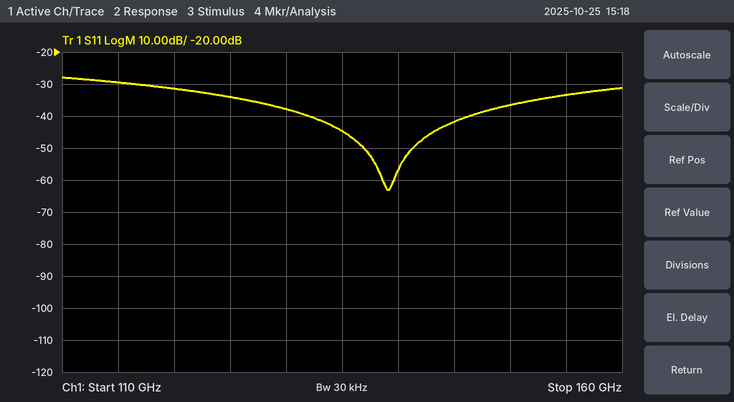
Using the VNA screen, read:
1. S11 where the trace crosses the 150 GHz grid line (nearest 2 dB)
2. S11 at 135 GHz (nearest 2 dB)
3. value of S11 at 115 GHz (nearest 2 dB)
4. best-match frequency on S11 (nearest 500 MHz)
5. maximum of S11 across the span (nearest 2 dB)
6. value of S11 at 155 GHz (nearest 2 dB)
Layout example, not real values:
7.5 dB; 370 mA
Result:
-36 dB; -44 dB; -30 dB; 139.0 GHz; -28 dB; -34 dB
